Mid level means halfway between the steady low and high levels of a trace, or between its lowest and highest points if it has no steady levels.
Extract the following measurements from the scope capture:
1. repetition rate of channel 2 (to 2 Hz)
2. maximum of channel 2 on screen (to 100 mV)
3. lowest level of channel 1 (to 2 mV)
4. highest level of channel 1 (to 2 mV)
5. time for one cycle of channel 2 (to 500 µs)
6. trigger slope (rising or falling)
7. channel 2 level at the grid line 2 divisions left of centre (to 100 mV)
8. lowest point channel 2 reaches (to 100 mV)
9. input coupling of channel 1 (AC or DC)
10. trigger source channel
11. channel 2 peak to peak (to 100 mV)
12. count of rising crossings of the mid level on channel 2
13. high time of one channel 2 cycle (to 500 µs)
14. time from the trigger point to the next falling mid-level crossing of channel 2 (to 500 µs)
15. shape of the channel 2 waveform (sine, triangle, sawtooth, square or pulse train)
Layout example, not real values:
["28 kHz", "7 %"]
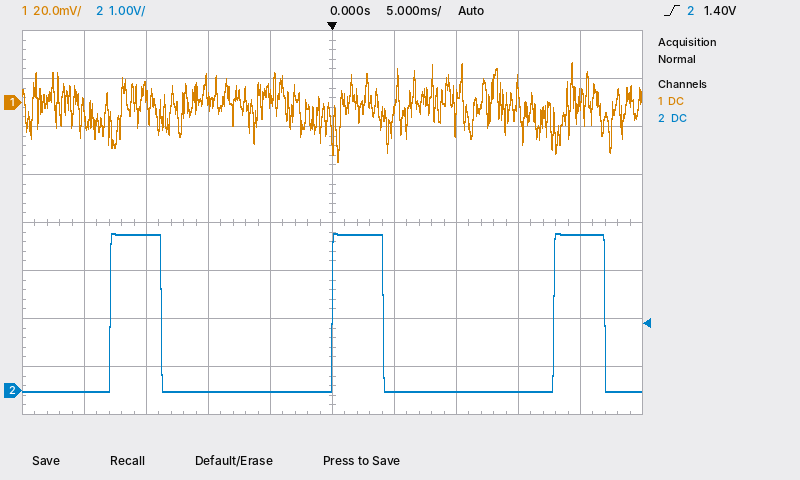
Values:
["56 Hz", "3.3 V", "-24 mV", "16 mV", "18.0 ms", "rising", "0.0 V", "0.0 V", "DC", "channel 2", "3.3 V", "3", "4.0 ms", "4.0 ms", "pulse train"]
